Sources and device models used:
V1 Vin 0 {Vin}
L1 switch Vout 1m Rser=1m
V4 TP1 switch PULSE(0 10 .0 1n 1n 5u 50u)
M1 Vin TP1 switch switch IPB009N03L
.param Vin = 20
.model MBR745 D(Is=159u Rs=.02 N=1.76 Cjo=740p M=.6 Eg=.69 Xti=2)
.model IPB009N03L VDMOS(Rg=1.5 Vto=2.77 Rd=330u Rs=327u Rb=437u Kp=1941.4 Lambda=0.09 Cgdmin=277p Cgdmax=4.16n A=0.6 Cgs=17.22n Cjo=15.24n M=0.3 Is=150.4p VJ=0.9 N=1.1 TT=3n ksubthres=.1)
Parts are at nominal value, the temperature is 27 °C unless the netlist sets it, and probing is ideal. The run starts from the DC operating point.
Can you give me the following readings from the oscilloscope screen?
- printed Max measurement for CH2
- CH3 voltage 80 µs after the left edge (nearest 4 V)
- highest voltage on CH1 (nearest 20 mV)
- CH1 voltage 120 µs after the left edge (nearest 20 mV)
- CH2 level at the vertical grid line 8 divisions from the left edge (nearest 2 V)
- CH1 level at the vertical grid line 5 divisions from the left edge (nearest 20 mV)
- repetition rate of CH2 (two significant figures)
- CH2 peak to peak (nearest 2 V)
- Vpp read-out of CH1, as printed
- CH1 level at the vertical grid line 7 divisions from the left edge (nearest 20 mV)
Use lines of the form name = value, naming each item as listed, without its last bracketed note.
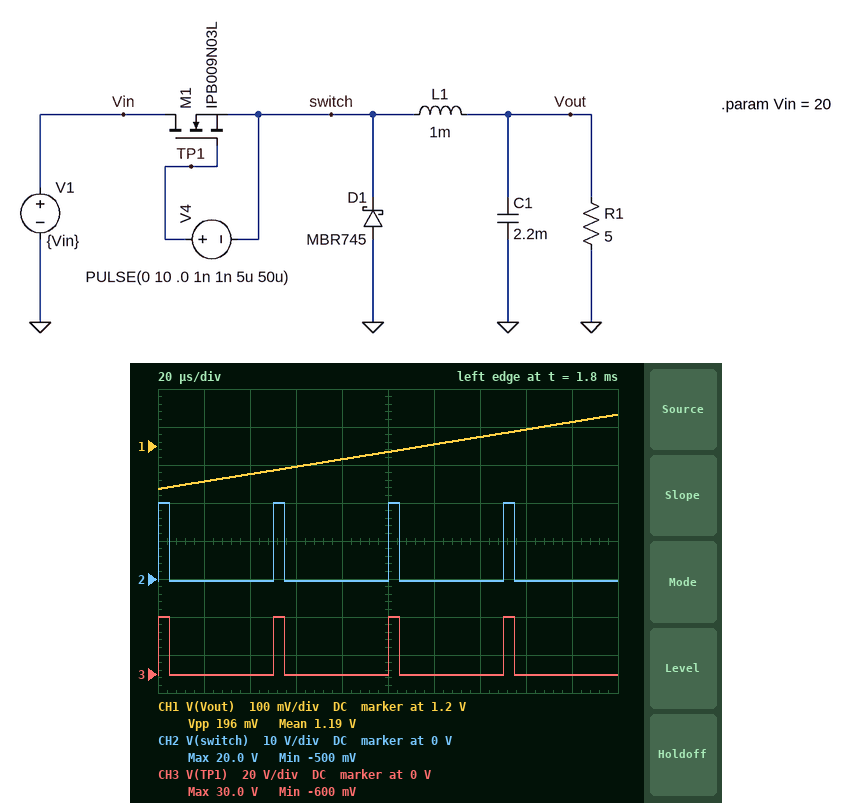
printed Max measurement for CH2 = 20.0 V
CH3 voltage 80 µs after the left edge = 0 V
highest voltage on CH1 = 1.28 V
CH1 voltage 120 µs after the left edge = 1.20 V
CH2 level at the vertical grid line 8 divisions from the left edge = 0 V
CH1 level at the vertical grid line 5 divisions from the left edge = 1.18 V
repetition rate of CH2 = 20 kHz
CH2 peak to peak = 20 V
Vpp read-out of CH1, as printed = 196 mV
CH1 level at the vertical grid line 7 divisions from the left edge = 1.22 V
